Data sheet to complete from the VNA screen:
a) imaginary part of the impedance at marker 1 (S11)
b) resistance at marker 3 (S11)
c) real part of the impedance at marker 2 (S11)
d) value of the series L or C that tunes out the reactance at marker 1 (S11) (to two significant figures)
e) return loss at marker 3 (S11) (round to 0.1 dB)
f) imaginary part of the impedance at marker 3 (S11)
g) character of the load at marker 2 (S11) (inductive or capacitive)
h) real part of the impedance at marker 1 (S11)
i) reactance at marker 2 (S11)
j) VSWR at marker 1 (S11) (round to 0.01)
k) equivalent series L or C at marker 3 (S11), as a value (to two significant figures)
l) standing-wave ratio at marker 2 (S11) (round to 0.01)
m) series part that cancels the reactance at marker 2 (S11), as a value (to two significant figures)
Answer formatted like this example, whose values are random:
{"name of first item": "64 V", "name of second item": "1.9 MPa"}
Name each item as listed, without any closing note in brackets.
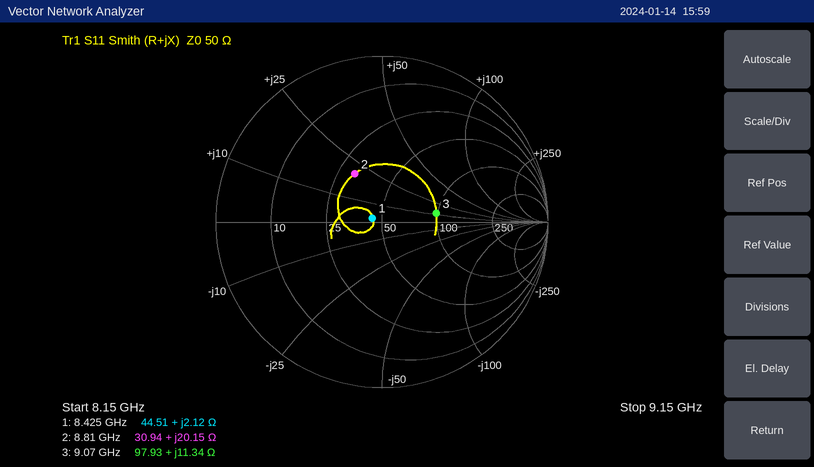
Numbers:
{"imaginary part of the impedance at marker 1": "+2.12 Ω", "resistance at marker 3": "97.93 Ω", "real part of the impedance at marker 2": "30.94 Ω", "value of the series L or C that tunes out the reactance at marker 1 (S11)": "8.9 pF", "return loss at marker 3 (S11)": "9.6 dB", "imaginary part of the impedance at marker 3": "+11.34 Ω", "character of the load at marker 2 (S11)": "inductive", "real part of the impedance at marker 1": "44.51 Ω", "reactance at marker 2": "+20.15 Ω", "VSWR at marker 1 (S11)": "1.13", "equivalent series L or C at marker 3 (S11), as a value": "200 pH", "standing-wave ratio at marker 2 (S11)": "2.00", "series part that cancels the reactance at marker 2 (S11), as a value": "900 fF"}
